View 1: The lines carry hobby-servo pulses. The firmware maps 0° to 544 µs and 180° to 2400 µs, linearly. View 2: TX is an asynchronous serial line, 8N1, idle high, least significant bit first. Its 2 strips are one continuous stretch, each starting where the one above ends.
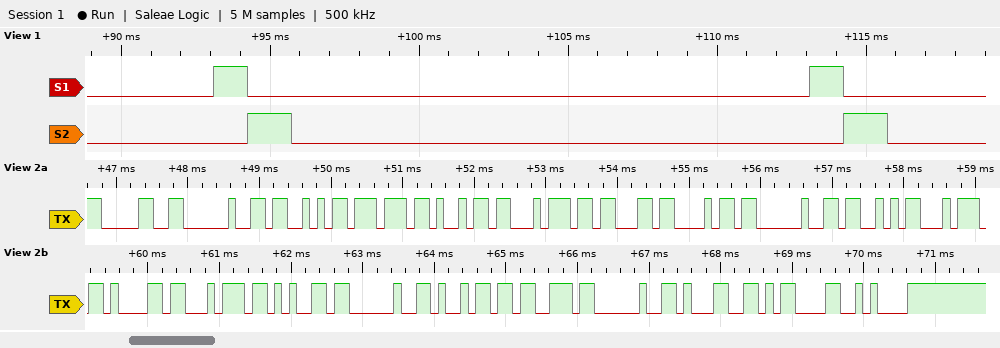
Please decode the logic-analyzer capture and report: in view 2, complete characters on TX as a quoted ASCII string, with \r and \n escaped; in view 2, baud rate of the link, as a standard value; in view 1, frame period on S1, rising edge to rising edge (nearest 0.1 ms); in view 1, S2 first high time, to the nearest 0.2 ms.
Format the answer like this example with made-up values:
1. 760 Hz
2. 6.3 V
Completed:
1. "0 Switch State is 1\r\n"
2. 9600 baud
3. 20.0 ms
4. 1.4 ms
